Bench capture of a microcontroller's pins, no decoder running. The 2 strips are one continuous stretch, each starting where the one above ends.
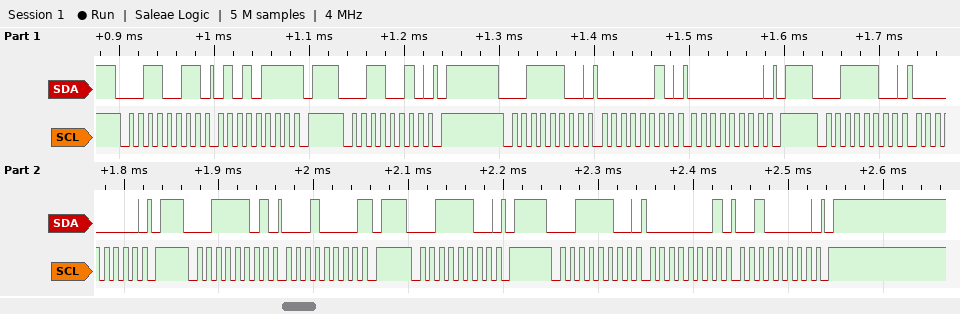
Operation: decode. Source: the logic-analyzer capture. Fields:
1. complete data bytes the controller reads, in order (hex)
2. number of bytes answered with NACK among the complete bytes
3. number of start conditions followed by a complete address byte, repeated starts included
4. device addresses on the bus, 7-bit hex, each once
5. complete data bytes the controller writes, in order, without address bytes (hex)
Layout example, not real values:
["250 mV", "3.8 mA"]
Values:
["57 10", "2", "7", "0x19 0x1E", "02 00 00 01 20"]
